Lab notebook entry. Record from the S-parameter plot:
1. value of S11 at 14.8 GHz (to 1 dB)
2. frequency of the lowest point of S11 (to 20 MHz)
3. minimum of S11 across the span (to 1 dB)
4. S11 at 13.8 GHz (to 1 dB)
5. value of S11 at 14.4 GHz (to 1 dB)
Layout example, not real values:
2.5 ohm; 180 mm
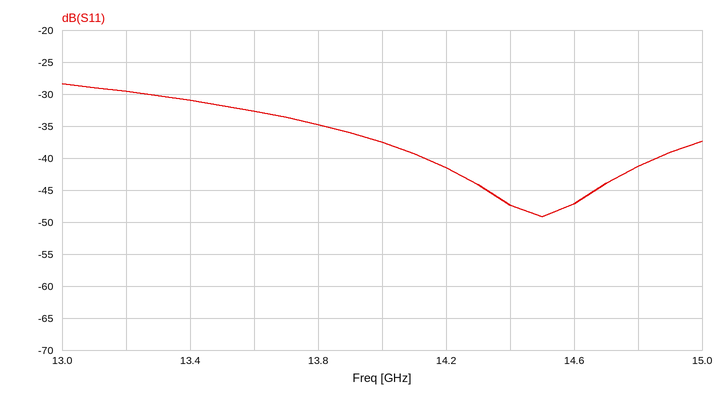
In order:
-41 dB; 14.50 GHz; -49 dB; -35 dB; -47 dB
